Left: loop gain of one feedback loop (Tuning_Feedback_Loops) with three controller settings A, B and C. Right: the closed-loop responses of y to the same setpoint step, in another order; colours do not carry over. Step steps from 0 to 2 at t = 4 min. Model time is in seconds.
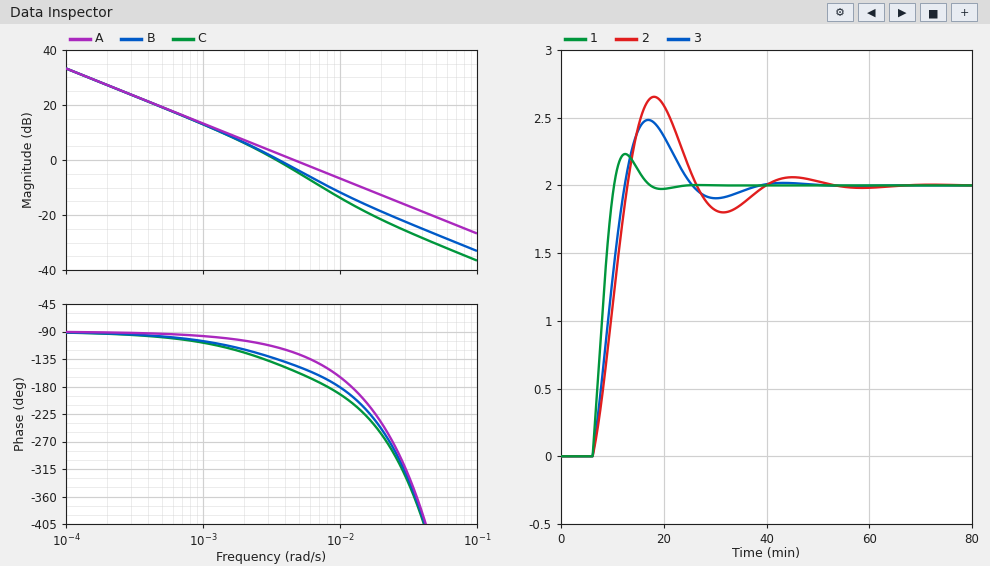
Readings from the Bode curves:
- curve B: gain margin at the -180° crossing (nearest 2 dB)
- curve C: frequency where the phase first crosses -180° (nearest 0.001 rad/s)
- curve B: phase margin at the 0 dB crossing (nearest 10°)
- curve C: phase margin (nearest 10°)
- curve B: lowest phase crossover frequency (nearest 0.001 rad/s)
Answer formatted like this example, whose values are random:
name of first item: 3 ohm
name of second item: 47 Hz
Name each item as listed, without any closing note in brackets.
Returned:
curve B: gain margin at the -180° crossing: 12 dB
curve C: frequency where the phase first crosses -180°: 0.008 rad/s
curve B: phase margin at the 0 dB crossing: 40°
curve C: phase margin: 40°
curve B: lowest phase crossover frequency: 0.010 rad/s
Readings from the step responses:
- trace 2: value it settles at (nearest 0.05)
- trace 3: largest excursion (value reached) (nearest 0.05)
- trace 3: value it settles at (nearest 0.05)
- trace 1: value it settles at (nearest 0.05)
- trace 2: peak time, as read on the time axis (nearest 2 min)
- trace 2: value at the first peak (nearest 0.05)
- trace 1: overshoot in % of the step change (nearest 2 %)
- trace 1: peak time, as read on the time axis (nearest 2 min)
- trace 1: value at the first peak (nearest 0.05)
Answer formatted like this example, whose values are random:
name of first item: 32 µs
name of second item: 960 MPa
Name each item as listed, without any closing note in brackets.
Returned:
trace 2: value it settles at: 2.00
trace 3: largest excursion (value reached): 2.50
trace 3: value it settles at: 2.00
trace 1: value it settles at: 2.00
trace 2: peak time, as read on the time axis: 18 min
trace 2: value at the first peak: 2.65
trace 1: overshoot in % of the step change: 12 %
trace 1: peak time, as read on the time axis: 12 min
trace 1: value at the first peak: 2.25
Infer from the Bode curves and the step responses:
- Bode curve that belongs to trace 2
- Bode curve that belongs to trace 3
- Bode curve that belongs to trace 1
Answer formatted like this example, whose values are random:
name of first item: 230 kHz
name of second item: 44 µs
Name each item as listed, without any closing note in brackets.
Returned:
Bode curve that belongs to trace 2: C
Bode curve that belongs to trace 3: B
Bode curve that belongs to trace 1: A
